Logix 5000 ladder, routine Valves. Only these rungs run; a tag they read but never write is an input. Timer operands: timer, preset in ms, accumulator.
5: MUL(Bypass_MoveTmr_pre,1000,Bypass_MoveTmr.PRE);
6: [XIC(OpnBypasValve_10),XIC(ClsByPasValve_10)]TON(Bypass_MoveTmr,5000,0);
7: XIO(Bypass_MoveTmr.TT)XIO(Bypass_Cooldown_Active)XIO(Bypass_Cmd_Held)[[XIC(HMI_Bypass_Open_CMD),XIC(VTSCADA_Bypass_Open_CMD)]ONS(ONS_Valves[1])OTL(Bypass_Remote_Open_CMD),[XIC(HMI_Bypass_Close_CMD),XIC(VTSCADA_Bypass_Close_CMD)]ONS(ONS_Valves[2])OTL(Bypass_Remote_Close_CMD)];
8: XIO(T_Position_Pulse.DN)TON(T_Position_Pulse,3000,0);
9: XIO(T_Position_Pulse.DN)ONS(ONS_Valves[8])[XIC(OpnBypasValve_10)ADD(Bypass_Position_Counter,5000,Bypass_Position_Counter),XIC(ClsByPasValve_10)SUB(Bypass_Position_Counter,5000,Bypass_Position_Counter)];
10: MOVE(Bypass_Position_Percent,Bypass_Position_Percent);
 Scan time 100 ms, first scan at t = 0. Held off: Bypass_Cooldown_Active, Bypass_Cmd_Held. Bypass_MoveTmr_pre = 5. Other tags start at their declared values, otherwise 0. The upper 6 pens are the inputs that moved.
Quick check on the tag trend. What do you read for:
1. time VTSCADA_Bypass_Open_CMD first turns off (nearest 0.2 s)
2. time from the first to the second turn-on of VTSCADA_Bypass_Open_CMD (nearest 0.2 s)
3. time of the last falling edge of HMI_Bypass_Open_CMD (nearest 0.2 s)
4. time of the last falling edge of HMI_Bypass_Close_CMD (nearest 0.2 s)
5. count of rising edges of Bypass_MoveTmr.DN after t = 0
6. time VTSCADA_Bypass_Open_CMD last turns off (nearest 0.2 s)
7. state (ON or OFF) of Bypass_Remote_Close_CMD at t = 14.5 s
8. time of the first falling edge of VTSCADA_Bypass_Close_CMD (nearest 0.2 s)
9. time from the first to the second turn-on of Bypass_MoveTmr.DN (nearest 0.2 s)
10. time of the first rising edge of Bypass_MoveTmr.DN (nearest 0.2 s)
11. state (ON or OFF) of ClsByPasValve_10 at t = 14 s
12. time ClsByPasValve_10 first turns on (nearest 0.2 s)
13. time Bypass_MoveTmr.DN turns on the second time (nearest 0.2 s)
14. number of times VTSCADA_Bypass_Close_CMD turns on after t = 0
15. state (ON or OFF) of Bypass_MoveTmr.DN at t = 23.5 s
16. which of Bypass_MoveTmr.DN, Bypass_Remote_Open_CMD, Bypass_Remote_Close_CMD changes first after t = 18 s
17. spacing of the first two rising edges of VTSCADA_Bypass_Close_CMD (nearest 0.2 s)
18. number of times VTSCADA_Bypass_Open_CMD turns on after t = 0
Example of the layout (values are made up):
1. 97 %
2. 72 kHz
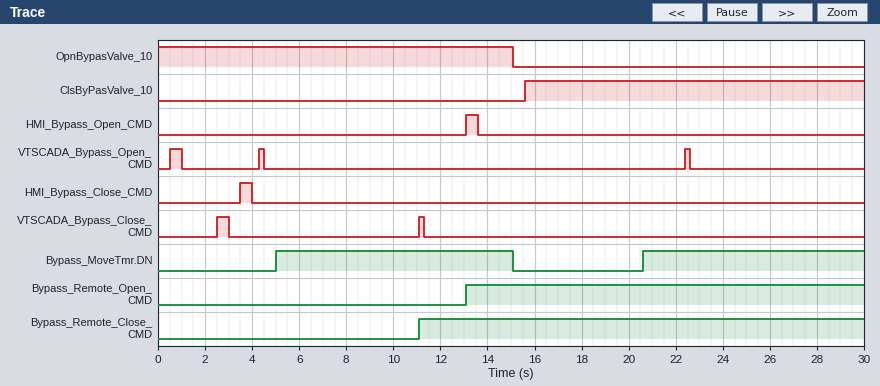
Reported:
1. 1.0 s
2. 3.8 s
3. 13.6 s
4. 4.0 s
5. 2
6. 22.6 s
7. ON
8. 3.0 s
9. 15.6 s
10. 5.0 s
11. OFF
12. 15.6 s
13. 20.6 s
14. 2
15. ON
16. Bypass_MoveTmr.DN
17. 8.6 s
18. 3
